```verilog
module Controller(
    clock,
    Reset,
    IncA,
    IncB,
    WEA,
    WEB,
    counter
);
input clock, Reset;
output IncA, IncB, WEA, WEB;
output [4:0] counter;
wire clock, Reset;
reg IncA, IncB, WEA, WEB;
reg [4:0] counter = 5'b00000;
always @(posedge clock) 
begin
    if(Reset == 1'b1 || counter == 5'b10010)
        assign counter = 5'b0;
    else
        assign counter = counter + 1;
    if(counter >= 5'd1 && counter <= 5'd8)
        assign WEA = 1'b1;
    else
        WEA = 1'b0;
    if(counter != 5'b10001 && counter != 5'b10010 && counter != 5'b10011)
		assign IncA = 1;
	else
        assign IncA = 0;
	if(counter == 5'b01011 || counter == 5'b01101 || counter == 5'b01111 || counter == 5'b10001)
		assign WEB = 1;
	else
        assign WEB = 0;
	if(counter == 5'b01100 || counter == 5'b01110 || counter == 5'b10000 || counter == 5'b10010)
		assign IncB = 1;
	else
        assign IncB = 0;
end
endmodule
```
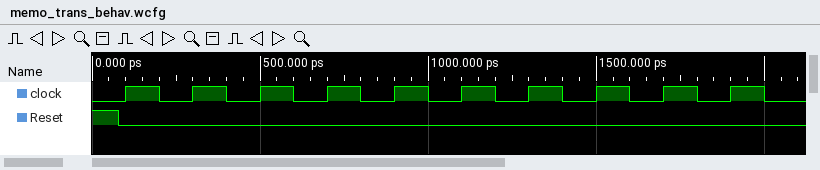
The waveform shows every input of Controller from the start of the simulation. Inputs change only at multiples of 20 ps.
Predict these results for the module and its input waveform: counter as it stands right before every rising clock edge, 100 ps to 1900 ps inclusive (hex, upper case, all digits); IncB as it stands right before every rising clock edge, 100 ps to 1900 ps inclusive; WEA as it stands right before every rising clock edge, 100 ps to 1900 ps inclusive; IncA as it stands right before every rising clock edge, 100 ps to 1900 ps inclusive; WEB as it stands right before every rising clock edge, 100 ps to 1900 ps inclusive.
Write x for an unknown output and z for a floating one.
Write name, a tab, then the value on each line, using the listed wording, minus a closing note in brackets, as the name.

counter as it stands right before every rising clock edge, 100 ps to 1900 ps inclusive	00, 01, 02, 03, 04, 05, 06, 07, 08, 09
IncB as it stands right before every rising clock edge, 100 ps to 1900 ps inclusive	x 0 0 0 0 0 0 0 0 0
WEA as it stands right before every rising clock edge, 100 ps to 1900 ps inclusive	x 1 1 1 1 1 1 1 1 1
IncA as it stands right before every rising clock edge, 100 ps to 1900 ps inclusive	x 1 1 1 1 1 1 1 1 1
WEB as it stands right before every rising clock edge, 100 ps to 1900 ps inclusive	x 0 0 0 0 0 0 0 0 0
